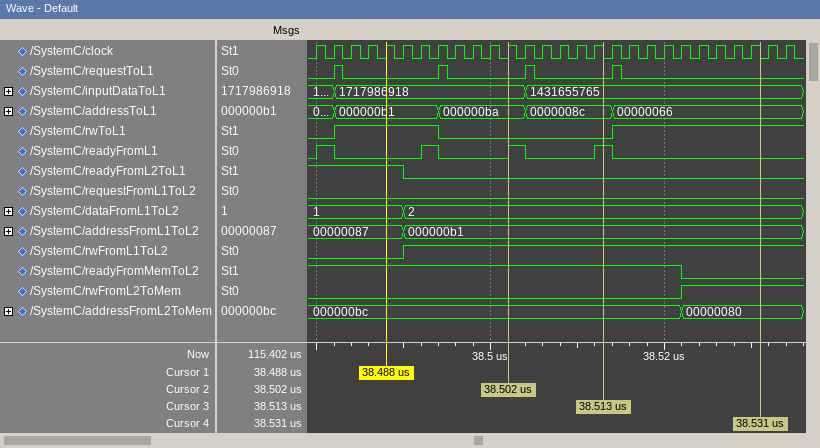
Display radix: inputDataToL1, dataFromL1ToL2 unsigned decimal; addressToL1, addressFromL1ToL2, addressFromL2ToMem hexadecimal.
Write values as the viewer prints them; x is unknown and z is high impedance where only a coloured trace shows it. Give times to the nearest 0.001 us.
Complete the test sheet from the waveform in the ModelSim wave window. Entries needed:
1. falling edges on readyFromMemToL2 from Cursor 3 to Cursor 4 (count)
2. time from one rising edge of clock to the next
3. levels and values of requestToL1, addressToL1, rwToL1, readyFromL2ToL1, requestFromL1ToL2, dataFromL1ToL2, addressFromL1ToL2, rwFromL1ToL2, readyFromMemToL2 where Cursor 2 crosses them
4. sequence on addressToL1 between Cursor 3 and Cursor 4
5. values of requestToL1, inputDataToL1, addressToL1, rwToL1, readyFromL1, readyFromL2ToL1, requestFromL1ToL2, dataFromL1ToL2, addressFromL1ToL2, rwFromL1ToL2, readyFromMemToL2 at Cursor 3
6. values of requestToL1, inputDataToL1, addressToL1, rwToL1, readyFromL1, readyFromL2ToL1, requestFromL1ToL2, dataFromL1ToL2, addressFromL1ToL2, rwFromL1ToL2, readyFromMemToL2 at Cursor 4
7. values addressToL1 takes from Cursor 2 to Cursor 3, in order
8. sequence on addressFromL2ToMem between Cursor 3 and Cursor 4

1
0.002 us
requestToL1=0, addressToL1=000000ba, rwToL1=0, readyFromL2ToL1=0, requestFromL1ToL2=0, dataFromL1ToL2=2, addressFromL1ToL2=000000b1, rwFromL1ToL2=1, readyFromMemToL2=1
0000008c, 00000066
requestToL1=0, inputDataToL1=1431655765, addressToL1=0000008c, rwToL1=0, readyFromL1=1, readyFromL2ToL1=0, requestFromL1ToL2=0, dataFromL1ToL2=2, addressFromL1ToL2=000000b1, rwFromL1ToL2=1, readyFromMemToL2=1
requestToL1=0, inputDataToL1=1431655765, addressToL1=00000066, rwToL1=1, readyFromL1=0, readyFromL2ToL1=0, requestFromL1ToL2=0, dataFromL1ToL2=2, addressFromL1ToL2=000000b1, rwFromL1ToL2=1, readyFromMemToL2=0
000000ba, 0000008c
000000bc, 00000080
